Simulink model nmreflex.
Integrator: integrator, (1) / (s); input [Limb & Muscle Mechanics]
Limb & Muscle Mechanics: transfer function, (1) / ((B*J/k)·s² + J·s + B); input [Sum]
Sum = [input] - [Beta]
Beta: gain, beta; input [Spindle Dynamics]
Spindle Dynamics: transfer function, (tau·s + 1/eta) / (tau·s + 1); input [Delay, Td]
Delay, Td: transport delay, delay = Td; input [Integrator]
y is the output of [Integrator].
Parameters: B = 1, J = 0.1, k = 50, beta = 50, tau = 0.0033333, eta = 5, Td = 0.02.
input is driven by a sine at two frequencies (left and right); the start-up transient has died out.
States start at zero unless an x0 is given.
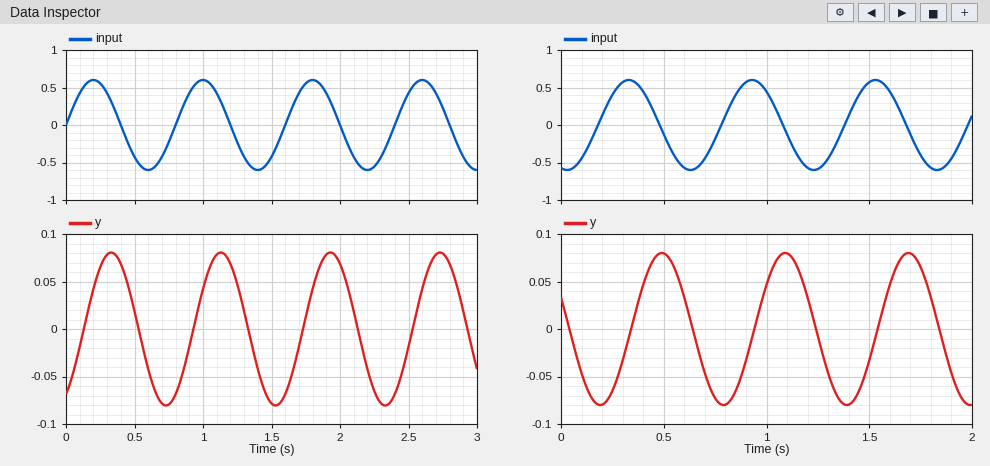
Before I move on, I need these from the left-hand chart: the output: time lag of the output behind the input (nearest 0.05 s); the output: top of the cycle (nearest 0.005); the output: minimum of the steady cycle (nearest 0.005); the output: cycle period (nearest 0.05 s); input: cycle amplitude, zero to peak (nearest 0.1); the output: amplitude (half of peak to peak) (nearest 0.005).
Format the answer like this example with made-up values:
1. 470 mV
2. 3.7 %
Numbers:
1. 0.15 s
2. 0.080
3. -0.080
4. 0.80 s
5. 0.6
6. 0.080
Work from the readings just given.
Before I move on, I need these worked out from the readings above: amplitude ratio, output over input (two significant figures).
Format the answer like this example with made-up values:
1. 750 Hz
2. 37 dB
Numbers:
1. 0.13
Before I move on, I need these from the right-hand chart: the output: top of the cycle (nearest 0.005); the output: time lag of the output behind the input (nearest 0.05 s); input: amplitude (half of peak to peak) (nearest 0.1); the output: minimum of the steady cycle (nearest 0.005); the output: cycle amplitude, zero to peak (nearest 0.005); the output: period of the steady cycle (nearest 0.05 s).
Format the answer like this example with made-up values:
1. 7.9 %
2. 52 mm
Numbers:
1. 0.080
2. 0.15 s
3. 0.6
4. -0.080
5. 0.080
6. 0.60 s
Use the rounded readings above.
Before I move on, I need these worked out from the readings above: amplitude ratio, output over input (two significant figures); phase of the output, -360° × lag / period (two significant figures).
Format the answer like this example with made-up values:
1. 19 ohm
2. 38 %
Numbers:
1. 0.13
2. -90°
